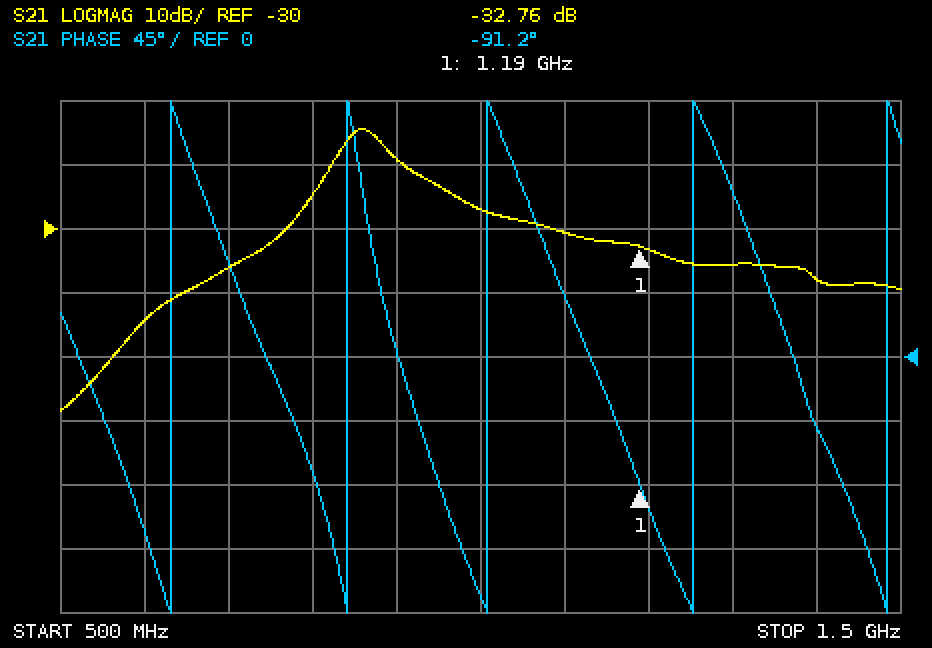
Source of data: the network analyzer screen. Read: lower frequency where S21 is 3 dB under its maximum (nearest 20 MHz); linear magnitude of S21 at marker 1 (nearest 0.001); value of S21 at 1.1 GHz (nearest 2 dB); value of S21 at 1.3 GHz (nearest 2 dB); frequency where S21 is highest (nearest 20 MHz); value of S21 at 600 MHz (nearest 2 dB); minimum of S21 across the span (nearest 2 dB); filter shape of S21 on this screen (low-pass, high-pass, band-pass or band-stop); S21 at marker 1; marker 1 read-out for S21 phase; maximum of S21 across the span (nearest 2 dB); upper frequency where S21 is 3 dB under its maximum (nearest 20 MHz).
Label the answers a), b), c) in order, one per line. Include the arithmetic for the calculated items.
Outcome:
a) 840 MHz
b) 10^(-32.76/20) ≈ 0.023
c) -30 dB
d) -36 dB
e) 860 MHz
f) -44 dB
g) -58 dB
h) band-pass
i) -32.76 dB
j) -91.2°
k) -14 dB
l) 880 MHz
